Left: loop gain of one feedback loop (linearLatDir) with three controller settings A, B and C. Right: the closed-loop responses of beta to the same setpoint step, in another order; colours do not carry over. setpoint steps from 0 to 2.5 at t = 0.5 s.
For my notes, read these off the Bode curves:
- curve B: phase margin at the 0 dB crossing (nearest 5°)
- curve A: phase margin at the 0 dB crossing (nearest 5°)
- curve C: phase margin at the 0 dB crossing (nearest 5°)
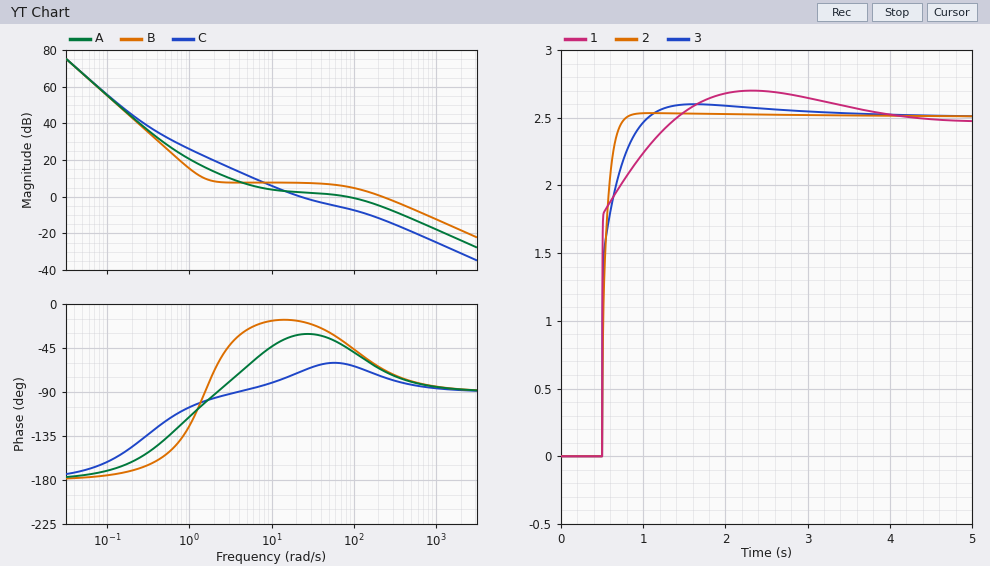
115°
135°
110°
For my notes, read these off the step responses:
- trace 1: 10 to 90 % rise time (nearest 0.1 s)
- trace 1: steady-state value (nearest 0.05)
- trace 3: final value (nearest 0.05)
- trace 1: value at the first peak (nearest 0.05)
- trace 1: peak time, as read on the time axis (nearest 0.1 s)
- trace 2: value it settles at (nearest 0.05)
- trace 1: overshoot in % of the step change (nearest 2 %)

0.5 s
2.50
2.50
2.70
2.3 s
2.50
8 %
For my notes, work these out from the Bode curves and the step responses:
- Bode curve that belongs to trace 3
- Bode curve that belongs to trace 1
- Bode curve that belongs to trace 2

A
B
C
